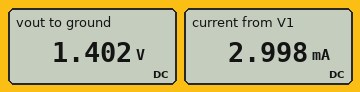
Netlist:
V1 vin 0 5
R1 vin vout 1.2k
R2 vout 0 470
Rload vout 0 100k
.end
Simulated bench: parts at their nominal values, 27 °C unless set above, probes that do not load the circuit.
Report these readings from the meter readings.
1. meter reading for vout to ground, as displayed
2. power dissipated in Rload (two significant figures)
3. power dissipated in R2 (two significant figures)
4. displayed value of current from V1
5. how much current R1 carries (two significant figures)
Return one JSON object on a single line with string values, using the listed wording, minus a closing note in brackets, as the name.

{"meter reading for vout to ground, as displayed": "1.402 V", "power dissipated in Rload": "20 µW", "power dissipated in R2": "4.2 mW", "displayed value of current from V1": "2.998 mA", "how much current R1 carries": "3.0 mA"}
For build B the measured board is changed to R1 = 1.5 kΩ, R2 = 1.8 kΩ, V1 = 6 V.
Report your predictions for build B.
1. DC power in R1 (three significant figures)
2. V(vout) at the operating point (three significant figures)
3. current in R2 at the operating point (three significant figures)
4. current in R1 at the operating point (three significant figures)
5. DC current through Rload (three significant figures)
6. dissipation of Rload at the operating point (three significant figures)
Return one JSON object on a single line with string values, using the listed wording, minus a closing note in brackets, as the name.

{"DC power in R1": "5.06 mW", "V(vout) at the operating point": "3.25 V", "current in R2 at the operating point": "1.80 mA", "current in R1 at the operating point": "1.84 mA", "DC current through Rload": "32.5 µA", "dissipation of Rload at the operating point": "105 µW"}
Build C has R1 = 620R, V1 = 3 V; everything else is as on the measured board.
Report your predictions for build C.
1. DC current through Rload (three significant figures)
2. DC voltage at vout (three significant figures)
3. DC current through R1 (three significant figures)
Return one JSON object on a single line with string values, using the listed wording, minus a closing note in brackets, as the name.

{"DC current through Rload": "12.9 µA", "DC voltage at vout": "1.29 V", "DC current through R1": "2.76 mA"}
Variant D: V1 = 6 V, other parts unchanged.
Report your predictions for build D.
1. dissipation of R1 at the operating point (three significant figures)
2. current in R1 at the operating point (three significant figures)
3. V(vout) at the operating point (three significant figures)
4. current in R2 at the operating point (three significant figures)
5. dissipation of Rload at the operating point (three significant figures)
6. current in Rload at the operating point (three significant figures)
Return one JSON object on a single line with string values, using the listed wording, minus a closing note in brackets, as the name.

{"dissipation of R1 at the operating point": "15.5 mW", "current in R1 at the operating point": "3.60 mA", "V(vout) at the operating point": "1.68 V", "current in R2 at the operating point": "3.58 mA", "dissipation of Rload at the operating point": "28.3 µW", "current in Rload at the operating point": "16.8 µA"}
